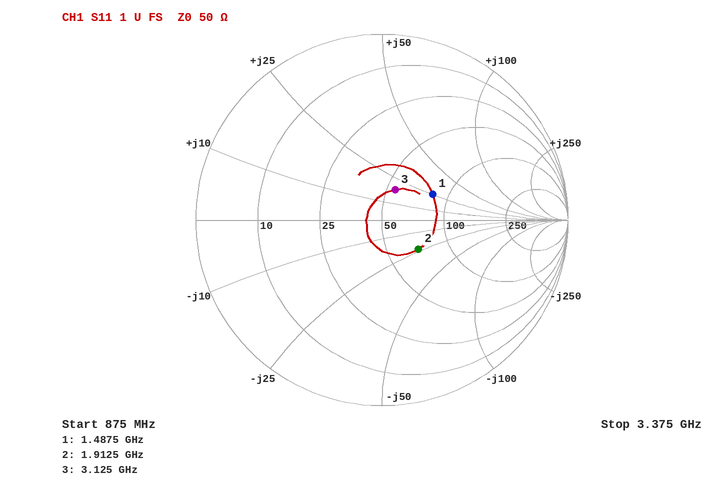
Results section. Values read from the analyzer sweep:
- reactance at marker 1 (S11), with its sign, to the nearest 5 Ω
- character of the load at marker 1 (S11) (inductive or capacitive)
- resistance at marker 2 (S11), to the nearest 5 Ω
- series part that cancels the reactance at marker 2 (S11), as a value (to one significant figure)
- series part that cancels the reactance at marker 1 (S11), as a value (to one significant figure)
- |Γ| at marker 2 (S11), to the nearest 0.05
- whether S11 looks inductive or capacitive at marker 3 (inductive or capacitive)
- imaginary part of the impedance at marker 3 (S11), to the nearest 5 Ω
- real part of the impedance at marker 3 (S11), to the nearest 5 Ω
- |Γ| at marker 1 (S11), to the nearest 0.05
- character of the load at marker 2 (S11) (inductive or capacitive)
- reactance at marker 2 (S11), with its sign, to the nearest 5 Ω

+25 Ω
inductive
70 Ω
2 nH
4 pF
0.25
inductive
+20 Ω
55 Ω
0.30
capacitive
-25 Ω
